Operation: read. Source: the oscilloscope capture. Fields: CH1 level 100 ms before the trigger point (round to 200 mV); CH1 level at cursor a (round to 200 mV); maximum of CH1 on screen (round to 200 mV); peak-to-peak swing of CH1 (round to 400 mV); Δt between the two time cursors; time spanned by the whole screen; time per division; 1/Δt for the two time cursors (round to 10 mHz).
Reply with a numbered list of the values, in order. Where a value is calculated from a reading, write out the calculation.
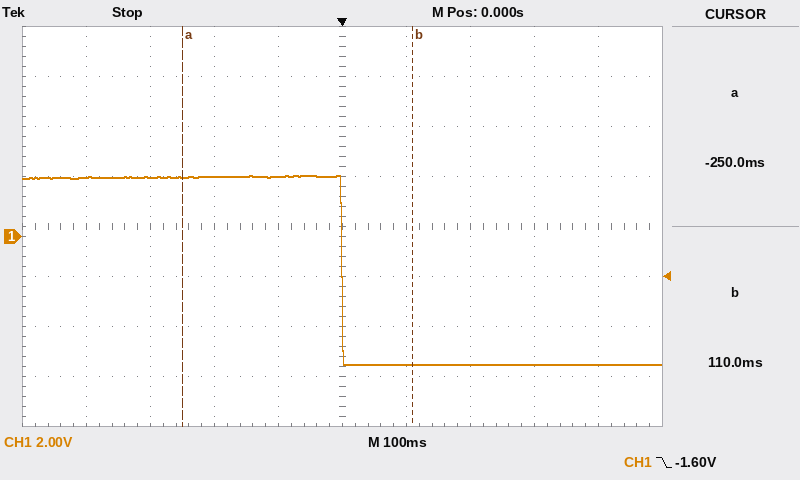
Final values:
1. 2.4 V
2. 2.4 V
3. 2.4 V
4. 7.6 V
5. 110 ms − (-250 ms) = 360 ms
6. 1 s
7. 100 ms
8. 1 / 360 ms ≈ 2.78 Hz
